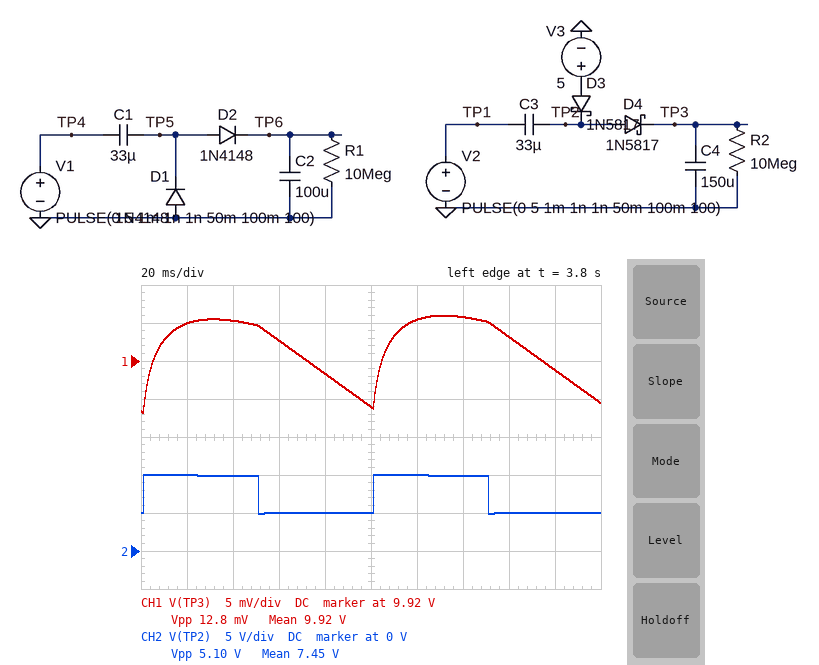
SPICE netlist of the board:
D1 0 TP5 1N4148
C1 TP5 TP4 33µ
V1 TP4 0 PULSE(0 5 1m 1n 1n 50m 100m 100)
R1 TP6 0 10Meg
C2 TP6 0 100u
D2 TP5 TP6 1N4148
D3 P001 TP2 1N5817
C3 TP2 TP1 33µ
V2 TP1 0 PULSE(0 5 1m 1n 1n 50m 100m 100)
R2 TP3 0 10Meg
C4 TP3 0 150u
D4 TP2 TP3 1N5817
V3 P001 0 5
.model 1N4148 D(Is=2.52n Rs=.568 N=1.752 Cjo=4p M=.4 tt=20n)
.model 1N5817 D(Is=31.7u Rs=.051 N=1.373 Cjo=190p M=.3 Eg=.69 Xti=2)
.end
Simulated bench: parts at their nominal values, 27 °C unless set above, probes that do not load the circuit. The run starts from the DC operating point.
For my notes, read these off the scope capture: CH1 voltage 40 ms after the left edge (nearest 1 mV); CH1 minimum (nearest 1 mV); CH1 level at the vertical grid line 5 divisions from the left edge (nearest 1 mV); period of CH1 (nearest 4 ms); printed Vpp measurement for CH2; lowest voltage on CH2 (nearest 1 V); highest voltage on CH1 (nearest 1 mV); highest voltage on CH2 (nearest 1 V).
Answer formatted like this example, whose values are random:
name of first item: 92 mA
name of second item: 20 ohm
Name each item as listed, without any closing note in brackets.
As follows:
CH1 voltage 40 ms after the left edge: 9.925 V
CH1 minimum: 9.913 V
CH1 level at the vertical grid line 5 divisions from the left edge: 9.914 V
period of CH1: 100 ms
printed Vpp measurement for CH2: 5.10 V
lowest voltage on CH2: 5 V
highest voltage on CH1: 9.926 V
highest voltage on CH2: 10 V
